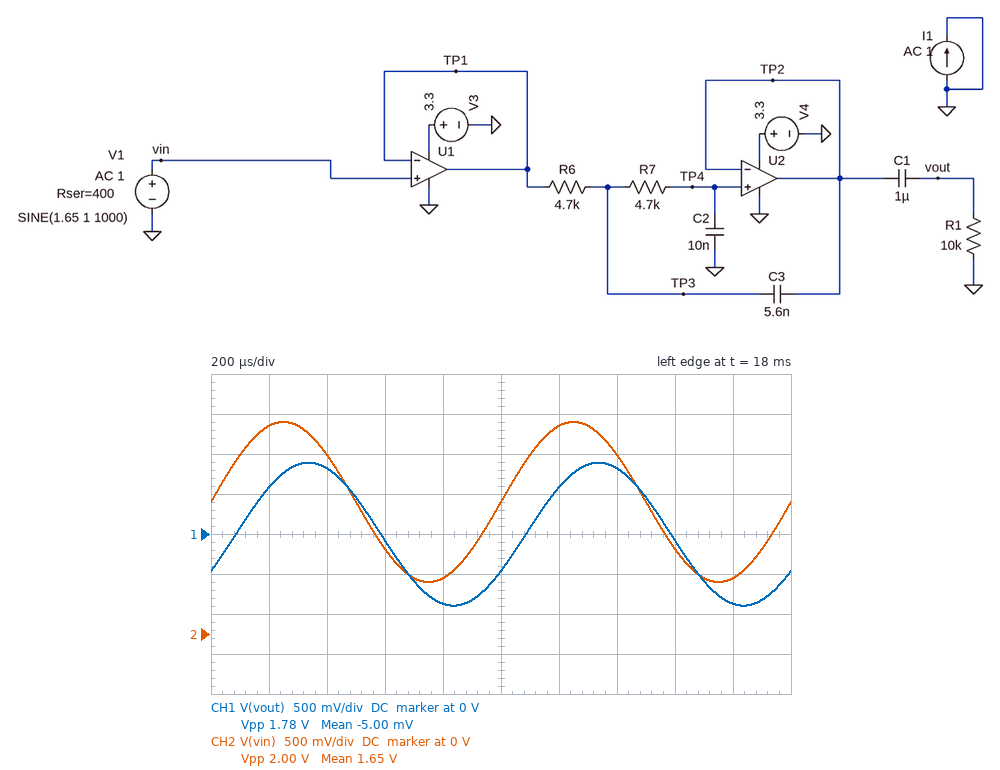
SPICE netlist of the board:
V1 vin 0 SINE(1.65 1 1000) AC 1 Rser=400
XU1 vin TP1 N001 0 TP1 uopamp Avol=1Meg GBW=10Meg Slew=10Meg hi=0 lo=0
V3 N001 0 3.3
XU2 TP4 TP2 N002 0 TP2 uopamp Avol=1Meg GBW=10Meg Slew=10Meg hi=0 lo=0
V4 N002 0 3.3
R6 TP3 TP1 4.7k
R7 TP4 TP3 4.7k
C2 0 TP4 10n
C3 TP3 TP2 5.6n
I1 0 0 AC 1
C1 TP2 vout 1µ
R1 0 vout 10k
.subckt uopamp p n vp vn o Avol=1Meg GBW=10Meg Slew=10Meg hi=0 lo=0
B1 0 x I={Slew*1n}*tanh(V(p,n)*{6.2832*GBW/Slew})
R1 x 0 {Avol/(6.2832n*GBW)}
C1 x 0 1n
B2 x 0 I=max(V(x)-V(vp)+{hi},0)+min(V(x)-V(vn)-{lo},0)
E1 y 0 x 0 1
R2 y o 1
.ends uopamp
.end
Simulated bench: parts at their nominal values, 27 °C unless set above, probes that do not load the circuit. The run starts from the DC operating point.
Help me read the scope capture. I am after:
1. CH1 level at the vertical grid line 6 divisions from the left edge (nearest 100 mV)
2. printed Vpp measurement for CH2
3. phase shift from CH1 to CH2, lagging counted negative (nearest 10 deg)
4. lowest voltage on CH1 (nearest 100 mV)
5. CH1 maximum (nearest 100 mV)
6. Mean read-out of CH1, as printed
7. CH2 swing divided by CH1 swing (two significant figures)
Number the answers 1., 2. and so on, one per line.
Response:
1. 600 mV
2. 2.00 V
3. 30 deg
4. -900 mV
5. 900 mV
6. -5.00 mV
7. 1.1
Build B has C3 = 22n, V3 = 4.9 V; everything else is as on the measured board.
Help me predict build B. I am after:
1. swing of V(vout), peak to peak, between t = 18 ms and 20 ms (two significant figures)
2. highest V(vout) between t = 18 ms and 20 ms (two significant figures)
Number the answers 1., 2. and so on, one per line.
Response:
1. 2.0 V
2. 1.0 V
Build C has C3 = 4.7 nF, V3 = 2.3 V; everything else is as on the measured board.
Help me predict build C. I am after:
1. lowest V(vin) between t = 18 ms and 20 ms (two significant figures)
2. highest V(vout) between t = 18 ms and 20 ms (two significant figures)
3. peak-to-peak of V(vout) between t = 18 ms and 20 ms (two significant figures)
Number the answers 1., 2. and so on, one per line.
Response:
1. 650 mV
2. 690 mV
3. 1.5 V
